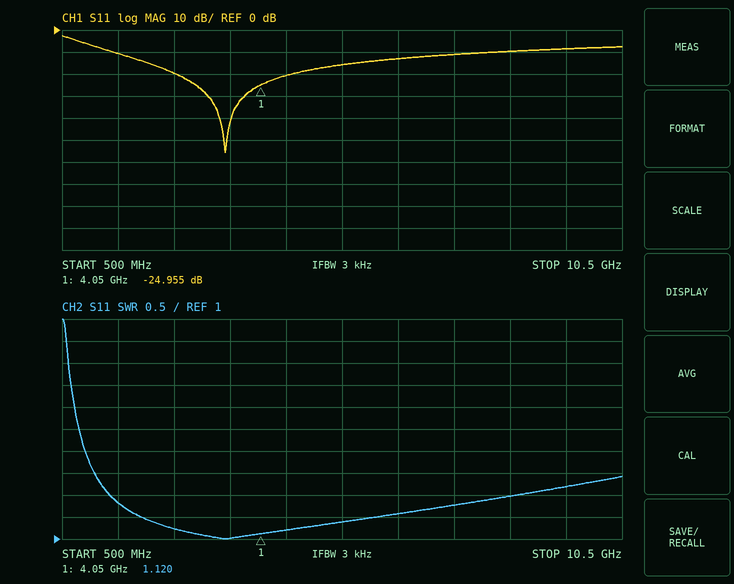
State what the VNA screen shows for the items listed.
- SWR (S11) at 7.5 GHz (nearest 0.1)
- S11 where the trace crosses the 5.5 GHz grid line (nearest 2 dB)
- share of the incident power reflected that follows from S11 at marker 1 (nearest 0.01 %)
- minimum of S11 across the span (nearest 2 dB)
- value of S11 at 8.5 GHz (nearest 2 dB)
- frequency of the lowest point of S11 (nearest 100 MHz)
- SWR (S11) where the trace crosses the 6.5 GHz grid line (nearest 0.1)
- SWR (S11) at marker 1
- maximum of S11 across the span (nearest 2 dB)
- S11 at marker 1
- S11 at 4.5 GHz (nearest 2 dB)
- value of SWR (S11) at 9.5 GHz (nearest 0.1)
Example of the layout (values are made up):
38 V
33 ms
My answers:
1.8
-16 dB
0.32 %
-56 dB
-10 dB
3.4 GHz
1.6
1.120
-2 dB
-24.955 dB
-20 dB
2.2
